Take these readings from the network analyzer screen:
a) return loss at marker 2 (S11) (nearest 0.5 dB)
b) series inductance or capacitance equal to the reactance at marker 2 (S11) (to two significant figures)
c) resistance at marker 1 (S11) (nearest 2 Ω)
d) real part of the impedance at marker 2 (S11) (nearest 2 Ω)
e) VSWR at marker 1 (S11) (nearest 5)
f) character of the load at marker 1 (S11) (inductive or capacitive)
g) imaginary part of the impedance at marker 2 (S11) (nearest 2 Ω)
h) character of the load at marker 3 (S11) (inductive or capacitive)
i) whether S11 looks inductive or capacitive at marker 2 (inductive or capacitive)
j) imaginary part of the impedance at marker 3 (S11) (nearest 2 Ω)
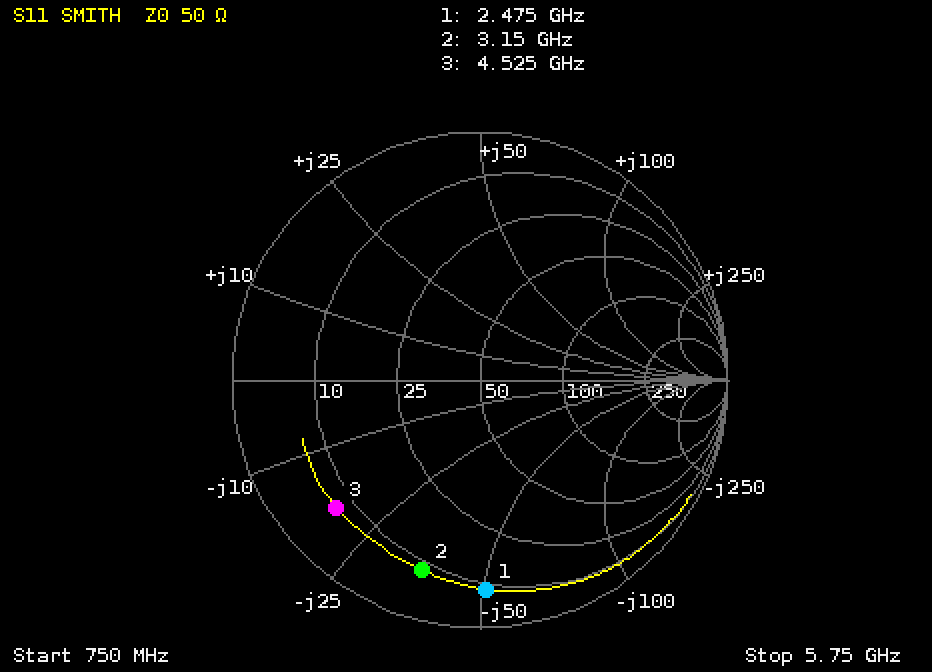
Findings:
2.0 dB
1.4 pF
8 Ω
8 Ω
10
capacitive
-36 Ω
capacitive
capacitive
-18 Ω
